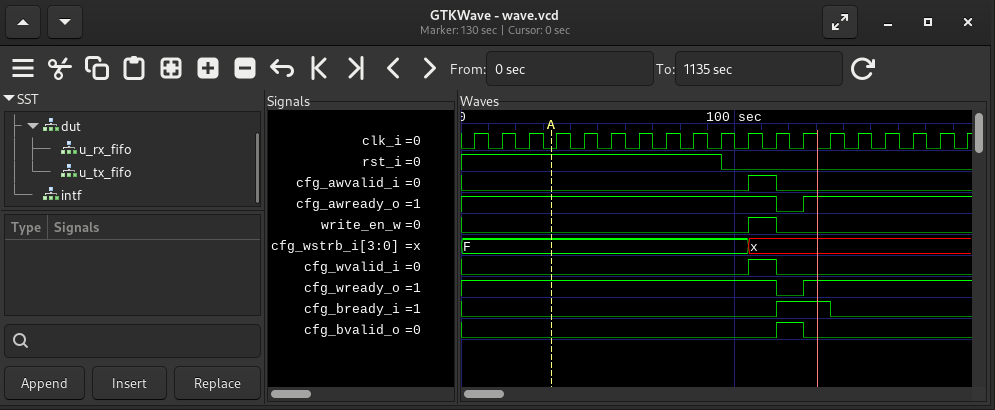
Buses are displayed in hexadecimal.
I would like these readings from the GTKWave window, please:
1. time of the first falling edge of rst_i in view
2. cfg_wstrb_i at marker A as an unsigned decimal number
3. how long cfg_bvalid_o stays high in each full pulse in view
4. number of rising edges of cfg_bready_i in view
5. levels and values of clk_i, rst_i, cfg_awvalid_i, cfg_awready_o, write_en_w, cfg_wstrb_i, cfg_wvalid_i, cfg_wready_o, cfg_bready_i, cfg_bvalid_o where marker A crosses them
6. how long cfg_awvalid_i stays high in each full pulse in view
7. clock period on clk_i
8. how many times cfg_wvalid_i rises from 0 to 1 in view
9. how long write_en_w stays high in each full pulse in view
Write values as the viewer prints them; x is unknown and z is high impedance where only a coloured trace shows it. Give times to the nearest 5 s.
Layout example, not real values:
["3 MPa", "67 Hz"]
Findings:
["95 s", "15", "10 s", "1", "clk_i=0, rst_i=1, cfg_awvalid_i=0, cfg_awready_o=1, write_en_w=0, cfg_wstrb_i=F, cfg_wvalid_i=0, cfg_wready_o=1, cfg_bready_i=0, cfg_bvalid_o=0", "10 s", "10 s", "1", "10 s"]
